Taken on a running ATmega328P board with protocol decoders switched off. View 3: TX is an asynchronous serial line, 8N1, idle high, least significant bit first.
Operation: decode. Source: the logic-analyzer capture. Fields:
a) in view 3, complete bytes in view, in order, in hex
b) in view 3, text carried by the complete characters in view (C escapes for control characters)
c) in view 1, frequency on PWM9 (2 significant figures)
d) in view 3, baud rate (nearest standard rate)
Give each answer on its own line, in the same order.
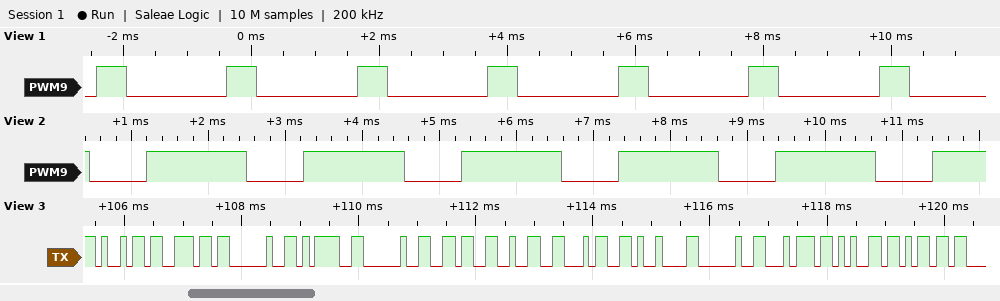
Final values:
0x69 0x6E 0x20 0x3D 0x20 0x36 0x32 0x34 0x09 0x20 0x74 0x65 0x6D
"in = 624\t tem"
490 Hz
9600 baud
